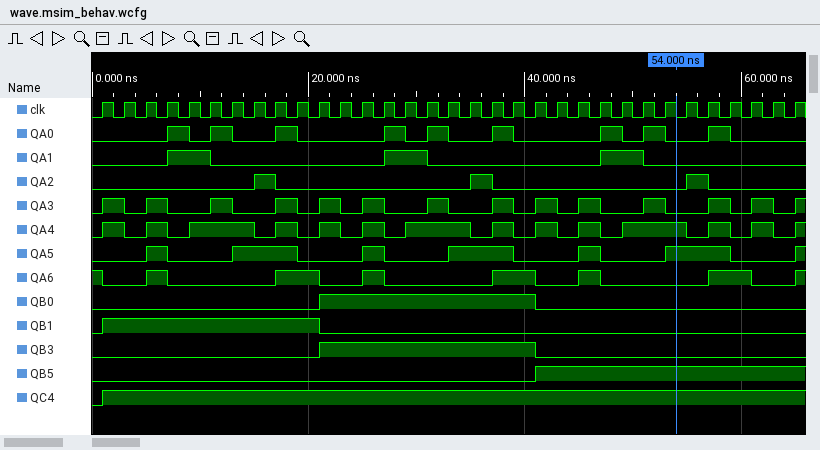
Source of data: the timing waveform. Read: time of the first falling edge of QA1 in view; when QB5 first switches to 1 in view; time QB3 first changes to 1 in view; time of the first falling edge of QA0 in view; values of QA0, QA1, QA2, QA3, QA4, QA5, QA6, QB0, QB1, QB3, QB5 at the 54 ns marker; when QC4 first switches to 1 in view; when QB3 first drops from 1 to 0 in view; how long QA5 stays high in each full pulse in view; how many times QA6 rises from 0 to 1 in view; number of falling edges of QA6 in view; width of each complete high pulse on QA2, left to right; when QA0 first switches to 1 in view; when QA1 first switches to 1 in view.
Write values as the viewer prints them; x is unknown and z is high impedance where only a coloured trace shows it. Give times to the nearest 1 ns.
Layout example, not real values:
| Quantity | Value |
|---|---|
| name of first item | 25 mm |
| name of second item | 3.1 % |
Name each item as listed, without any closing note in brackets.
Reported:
| Quantity | Value |
|---|---|
| time of the first falling edge of QA1 in view | 11 ns |
| when QB5 first switches to 1 in view | 41 ns |
| time QB3 first changes to 1 in view | 21 ns |
| time of the first falling edge of QA0 in view | 9 ns |
| values of QA0, QA1, QA2, QA3, QA4, QA5, QA6, QB0, QB1, QB3, QB5 at the 54 ns marker | QA0=0, QA1=0, QA2=0, QA3=0, QA4=1, QA5=1, QA6=0, QB0=0, QB1=0, QB3=0, QB5=1 |
| when QC4 first switches to 1 in view | 1 ns |
| when QB3 first drops from 1 to 0 in view | 41 ns |
| how long QA5 stays high in each full pulse in view | 2 ns, 6 ns, 2 ns, 6 ns, 2 ns, 6 ns |
| how many times QA6 rises from 0 to 1 in view | 7 |
| number of falling edges of QA6 in view | 7 |
| width of each complete high pulse on QA2, left to right | 2 ns, 2 ns, 2 ns |
| when QA0 first switches to 1 in view | 7 ns |
| when QA1 first switches to 1 in view | 7 ns |
